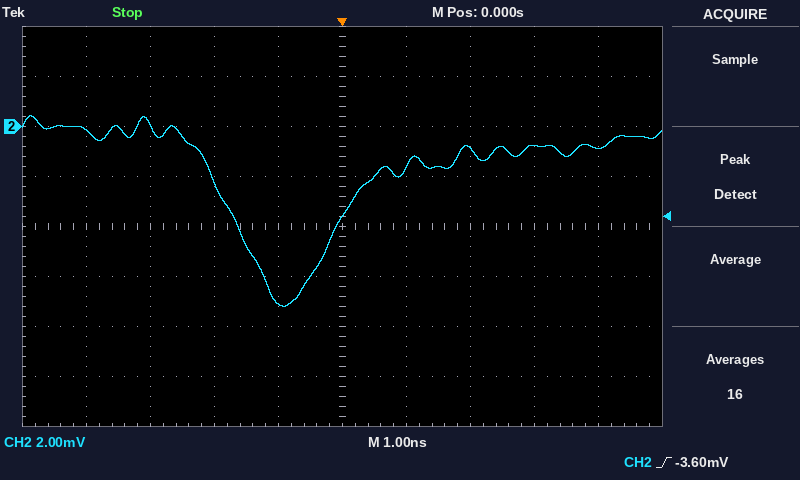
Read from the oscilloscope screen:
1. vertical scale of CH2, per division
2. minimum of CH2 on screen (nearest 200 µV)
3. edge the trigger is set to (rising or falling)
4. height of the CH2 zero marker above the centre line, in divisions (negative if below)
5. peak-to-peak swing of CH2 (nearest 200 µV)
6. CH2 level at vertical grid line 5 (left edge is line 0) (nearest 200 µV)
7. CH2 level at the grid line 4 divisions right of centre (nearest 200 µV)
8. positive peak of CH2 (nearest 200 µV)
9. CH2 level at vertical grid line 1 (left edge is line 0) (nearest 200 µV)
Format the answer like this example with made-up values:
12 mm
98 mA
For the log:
2 mV
-7.2 mV
rising
+2.0 div
7.6 mV
-3.6 mV
-800 µV
400 µV
-200 µV
